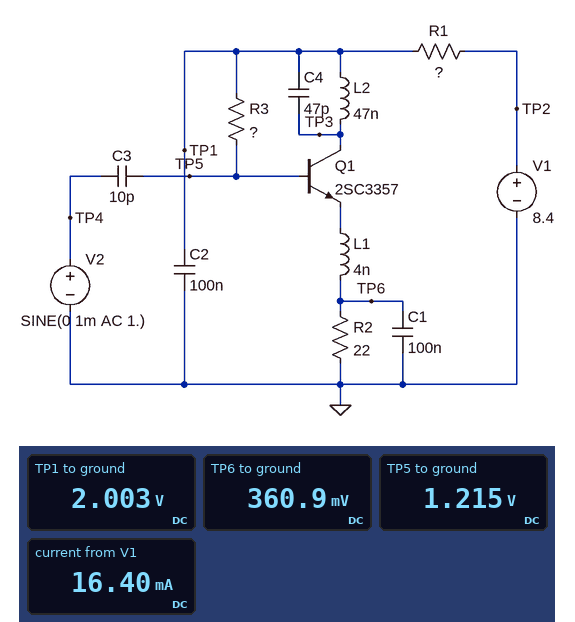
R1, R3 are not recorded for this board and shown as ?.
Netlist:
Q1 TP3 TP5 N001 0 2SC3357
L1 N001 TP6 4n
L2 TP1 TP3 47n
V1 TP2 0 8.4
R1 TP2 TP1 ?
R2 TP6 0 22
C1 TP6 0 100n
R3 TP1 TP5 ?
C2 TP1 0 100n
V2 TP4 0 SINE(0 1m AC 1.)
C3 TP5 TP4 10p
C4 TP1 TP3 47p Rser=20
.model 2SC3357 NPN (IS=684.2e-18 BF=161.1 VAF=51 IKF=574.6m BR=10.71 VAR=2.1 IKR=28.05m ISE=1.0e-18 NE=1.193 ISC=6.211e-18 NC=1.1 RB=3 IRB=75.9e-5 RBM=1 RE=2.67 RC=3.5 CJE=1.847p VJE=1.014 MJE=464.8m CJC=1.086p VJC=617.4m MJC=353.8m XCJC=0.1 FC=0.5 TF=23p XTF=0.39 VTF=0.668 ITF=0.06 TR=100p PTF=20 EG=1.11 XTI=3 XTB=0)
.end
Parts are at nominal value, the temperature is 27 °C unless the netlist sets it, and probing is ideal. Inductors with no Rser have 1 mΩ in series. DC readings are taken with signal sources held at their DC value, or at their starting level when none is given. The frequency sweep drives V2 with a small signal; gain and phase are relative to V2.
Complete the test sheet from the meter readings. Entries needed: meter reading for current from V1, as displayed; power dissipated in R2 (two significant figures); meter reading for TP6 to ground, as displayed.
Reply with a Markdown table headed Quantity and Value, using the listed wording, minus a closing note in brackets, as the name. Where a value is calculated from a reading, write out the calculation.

| Quantity | Value |
|---|---|
| meter reading for current from V1, as displayed | 16.40 mA |
| power dissipated in R2 | (360.9 mV)^2 / 22 Ω = 5.9 mW |
| meter reading for TP6 to ground, as displayed | 360.9 mV |
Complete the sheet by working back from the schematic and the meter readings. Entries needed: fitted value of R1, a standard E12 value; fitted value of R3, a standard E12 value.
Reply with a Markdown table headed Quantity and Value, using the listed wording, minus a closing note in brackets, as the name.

| Quantity | Value |
|---|---|
| fitted value of R1, a standard E12 value | 390 Ω |
| fitted value of R3, a standard E12 value | 4.7 kΩ |
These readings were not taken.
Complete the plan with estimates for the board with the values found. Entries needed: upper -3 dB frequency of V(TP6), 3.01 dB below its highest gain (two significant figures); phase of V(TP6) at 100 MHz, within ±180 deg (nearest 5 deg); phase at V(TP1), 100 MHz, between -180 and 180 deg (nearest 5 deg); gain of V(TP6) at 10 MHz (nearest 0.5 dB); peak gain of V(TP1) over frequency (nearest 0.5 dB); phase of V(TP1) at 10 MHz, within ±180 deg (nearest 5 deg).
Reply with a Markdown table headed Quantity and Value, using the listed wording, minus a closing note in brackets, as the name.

| Quantity | Value |
|---|---|
| upper -3 dB frequency of V(TP6), 3.01 dB below its highest gain | 28 MHz |
| phase of V(TP6) at 100 MHz, within ±180 deg | -110 deg |
| phase at V(TP1), 100 MHz, between -180 and 180 deg | 70 deg |
| gain of V(TP6) at 10 MHz | -42.0 dB |
| peak gain of V(TP1) over frequency | -41.5 dB |
| phase of V(TP1) at 10 MHz, within ±180 deg | 155 deg |
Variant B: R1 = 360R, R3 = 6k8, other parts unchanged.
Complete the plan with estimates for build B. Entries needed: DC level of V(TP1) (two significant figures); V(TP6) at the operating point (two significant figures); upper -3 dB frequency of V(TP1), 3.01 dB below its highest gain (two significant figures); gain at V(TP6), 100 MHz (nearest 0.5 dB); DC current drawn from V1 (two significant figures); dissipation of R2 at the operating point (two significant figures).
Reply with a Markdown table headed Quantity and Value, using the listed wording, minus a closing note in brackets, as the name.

| Quantity | Value |
|---|---|
| DC level of V(TP1) | 2.4 V |
| V(TP6) at the operating point | 370 mV |
| upper -3 dB frequency of V(TP1), 3.01 dB below its highest gain | 27 MHz |
| gain at V(TP6), 100 MHz | -57.5 dB |
| DC current drawn from V1 | 17 mA |
| dissipation of R2 at the operating point | 6.2 mW |
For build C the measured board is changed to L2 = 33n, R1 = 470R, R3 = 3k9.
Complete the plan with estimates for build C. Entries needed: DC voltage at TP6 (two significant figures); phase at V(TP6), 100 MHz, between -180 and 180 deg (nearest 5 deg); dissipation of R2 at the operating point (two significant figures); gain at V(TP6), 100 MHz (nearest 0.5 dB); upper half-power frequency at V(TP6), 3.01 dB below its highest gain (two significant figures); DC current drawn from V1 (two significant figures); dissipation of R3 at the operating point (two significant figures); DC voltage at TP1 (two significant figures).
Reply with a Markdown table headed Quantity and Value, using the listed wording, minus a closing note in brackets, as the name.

| Quantity | Value |
|---|---|
| DC voltage at TP6 | 310 mV |
| phase at V(TP6), 100 MHz, between -180 and 180 deg | -110 deg |
| dissipation of R2 at the operating point | 4.4 mW |
| gain at V(TP6), 100 MHz | -56.5 dB |
| upper half-power frequency at V(TP6), 3.01 dB below its highest gain | 26 MHz |
| DC current drawn from V1 | 14 mA |
| dissipation of R3 at the operating point | 82 µW |
| DC voltage at TP1 | 1.7 V |
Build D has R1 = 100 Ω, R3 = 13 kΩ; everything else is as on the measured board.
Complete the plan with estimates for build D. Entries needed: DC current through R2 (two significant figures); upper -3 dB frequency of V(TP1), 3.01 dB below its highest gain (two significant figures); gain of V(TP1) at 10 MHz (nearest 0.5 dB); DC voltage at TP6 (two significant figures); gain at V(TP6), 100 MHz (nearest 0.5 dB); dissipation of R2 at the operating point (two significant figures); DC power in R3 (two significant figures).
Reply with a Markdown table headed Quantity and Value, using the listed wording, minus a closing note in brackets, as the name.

| Quantity | Value |
|---|---|
| DC current through R2 | 30 mA |
| upper -3 dB frequency of V(TP1), 3.01 dB below its highest gain | 32 MHz |
| gain of V(TP1) at 10 MHz | -41.5 dB |
| DC voltage at TP6 | 660 mV |
| gain at V(TP6), 100 MHz | -55.5 dB |
| dissipation of R2 at the operating point | 20 mW |
| DC power in R3 | 1.1 mW |
